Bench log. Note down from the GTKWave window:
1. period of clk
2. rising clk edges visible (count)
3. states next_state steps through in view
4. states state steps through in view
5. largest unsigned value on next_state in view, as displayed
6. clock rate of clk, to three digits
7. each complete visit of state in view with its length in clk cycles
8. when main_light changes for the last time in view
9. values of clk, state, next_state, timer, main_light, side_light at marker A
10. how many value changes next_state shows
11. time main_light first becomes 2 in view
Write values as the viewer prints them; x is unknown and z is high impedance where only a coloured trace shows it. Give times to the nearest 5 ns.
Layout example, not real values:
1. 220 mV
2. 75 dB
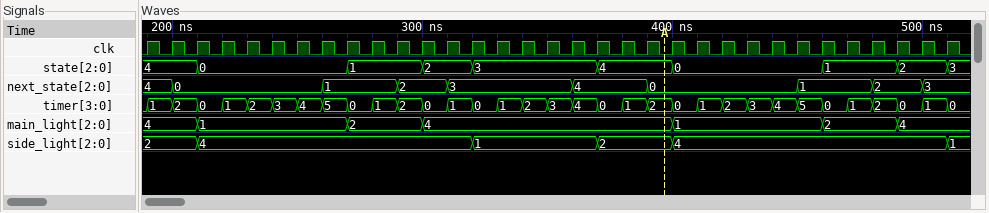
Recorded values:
1. 10 ns
2. 33
3. 4, 0, 1, 2, 3, 4, 0, 1, 2, 3
4. 4, 0, 1, 2, 3, 4, 0, 1, 2, 3
5. 4
6. 100 MHz
7. 0: 6, 1: 3, 2: 2, 3: 5, 4: 3, 0: 6, 1: 3, 2: 2
8. 490 ns
9. clk=0, state=4, next_state=0, timer=2, main_light=4, side_light=2
10. 9
11. 270 ns
